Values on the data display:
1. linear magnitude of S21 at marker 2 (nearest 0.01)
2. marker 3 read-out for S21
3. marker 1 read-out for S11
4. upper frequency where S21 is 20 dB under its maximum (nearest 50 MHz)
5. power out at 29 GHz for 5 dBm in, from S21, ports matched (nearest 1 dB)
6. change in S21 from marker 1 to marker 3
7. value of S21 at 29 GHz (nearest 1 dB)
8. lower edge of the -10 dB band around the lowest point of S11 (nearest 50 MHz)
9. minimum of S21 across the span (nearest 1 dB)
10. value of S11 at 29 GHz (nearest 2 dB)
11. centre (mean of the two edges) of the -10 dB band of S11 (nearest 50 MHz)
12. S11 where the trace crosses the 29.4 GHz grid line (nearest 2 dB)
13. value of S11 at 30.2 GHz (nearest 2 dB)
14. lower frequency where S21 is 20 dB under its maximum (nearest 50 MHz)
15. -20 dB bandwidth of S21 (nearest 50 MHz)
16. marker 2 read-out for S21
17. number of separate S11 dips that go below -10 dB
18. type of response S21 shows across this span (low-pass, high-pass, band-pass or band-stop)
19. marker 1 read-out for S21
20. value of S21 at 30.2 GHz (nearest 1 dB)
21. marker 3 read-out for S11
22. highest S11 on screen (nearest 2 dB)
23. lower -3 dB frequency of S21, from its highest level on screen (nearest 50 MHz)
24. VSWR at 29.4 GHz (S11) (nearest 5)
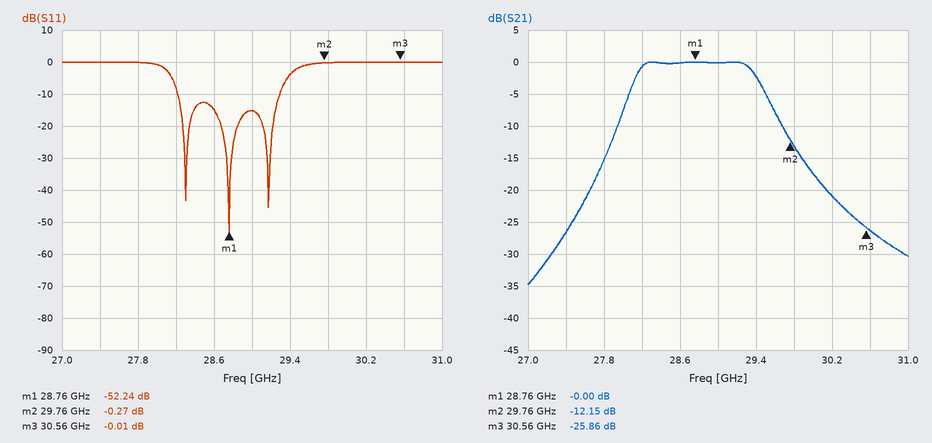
0.25
-25.86 dB
-52.24 dB
30.15 GHz
5 dBm
-25.86 dB
0 dB
28.20 GHz
-35 dB
-16 dB
28.75 GHz
-4 dB
0 dB
27.65 GHz
2.50 GHz
-12.15 dB
3
band-pass
-0.00 dB
-21 dB
-0.01 dB
0 dB
28.10 GHz
5
